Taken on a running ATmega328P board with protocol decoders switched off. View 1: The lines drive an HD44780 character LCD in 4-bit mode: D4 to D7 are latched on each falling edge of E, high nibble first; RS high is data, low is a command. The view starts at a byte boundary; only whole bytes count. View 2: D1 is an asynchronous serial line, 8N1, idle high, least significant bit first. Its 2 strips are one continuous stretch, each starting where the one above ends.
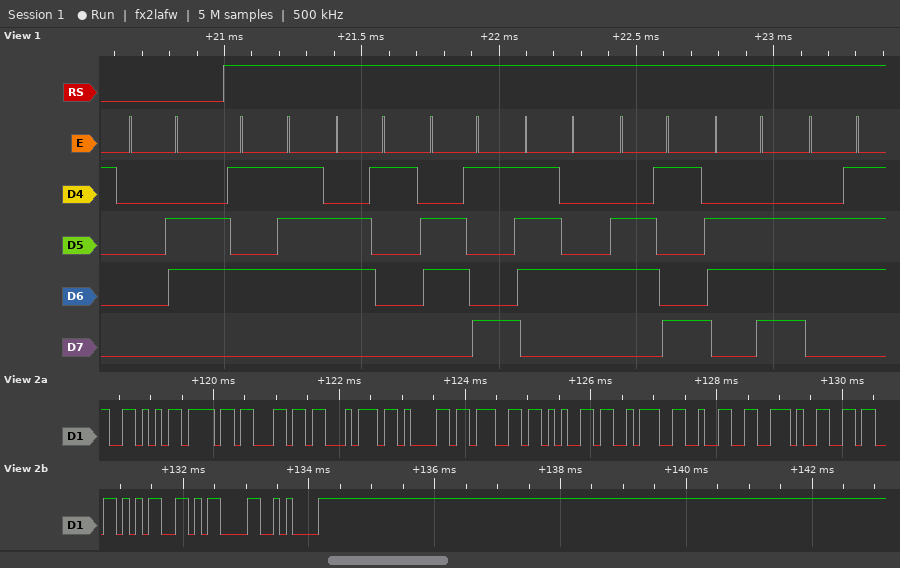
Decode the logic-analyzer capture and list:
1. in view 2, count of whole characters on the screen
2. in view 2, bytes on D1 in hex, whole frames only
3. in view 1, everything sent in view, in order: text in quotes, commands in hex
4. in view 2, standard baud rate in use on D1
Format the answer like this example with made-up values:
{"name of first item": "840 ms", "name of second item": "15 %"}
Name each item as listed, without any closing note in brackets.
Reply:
{"in view 2, count of whole characters on the screen": "14", "in view 2, bytes on D1 in hex, whole frames only": "56 6F 6C 74 61 67 65 3A 32 2E 36 35 0D 0A", "in view 1, everything sent in view, in order: text in quotes, commands in hex": "0x06 \"Waiting\"", "in view 2, standard baud rate in use on D1": "9600 baud"}
